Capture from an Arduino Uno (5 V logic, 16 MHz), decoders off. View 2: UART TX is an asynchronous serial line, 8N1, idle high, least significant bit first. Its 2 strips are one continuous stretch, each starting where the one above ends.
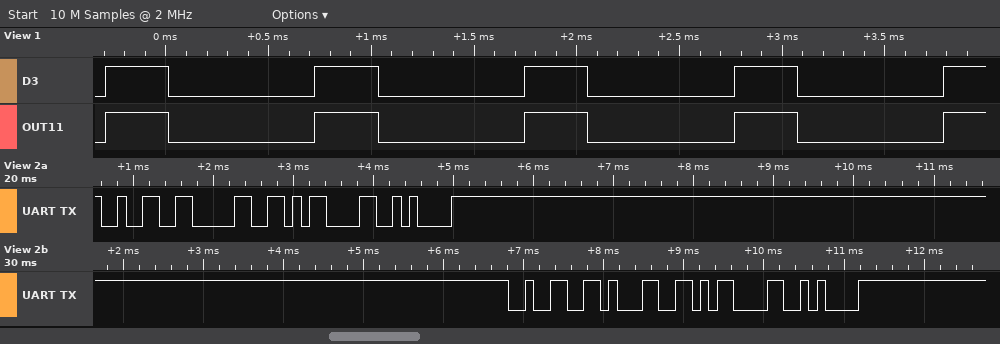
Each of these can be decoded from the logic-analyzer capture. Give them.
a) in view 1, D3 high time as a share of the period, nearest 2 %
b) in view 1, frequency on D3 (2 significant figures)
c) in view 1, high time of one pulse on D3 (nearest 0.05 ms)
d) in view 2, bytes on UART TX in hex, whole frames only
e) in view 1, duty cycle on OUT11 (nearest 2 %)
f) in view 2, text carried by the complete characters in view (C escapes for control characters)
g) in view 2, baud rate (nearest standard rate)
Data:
30 %
980 Hz
0.30 ms
32 30 0D 0A 32 31 0D 0A
30 %
"20\r\n21\r\n"
9600 baud
